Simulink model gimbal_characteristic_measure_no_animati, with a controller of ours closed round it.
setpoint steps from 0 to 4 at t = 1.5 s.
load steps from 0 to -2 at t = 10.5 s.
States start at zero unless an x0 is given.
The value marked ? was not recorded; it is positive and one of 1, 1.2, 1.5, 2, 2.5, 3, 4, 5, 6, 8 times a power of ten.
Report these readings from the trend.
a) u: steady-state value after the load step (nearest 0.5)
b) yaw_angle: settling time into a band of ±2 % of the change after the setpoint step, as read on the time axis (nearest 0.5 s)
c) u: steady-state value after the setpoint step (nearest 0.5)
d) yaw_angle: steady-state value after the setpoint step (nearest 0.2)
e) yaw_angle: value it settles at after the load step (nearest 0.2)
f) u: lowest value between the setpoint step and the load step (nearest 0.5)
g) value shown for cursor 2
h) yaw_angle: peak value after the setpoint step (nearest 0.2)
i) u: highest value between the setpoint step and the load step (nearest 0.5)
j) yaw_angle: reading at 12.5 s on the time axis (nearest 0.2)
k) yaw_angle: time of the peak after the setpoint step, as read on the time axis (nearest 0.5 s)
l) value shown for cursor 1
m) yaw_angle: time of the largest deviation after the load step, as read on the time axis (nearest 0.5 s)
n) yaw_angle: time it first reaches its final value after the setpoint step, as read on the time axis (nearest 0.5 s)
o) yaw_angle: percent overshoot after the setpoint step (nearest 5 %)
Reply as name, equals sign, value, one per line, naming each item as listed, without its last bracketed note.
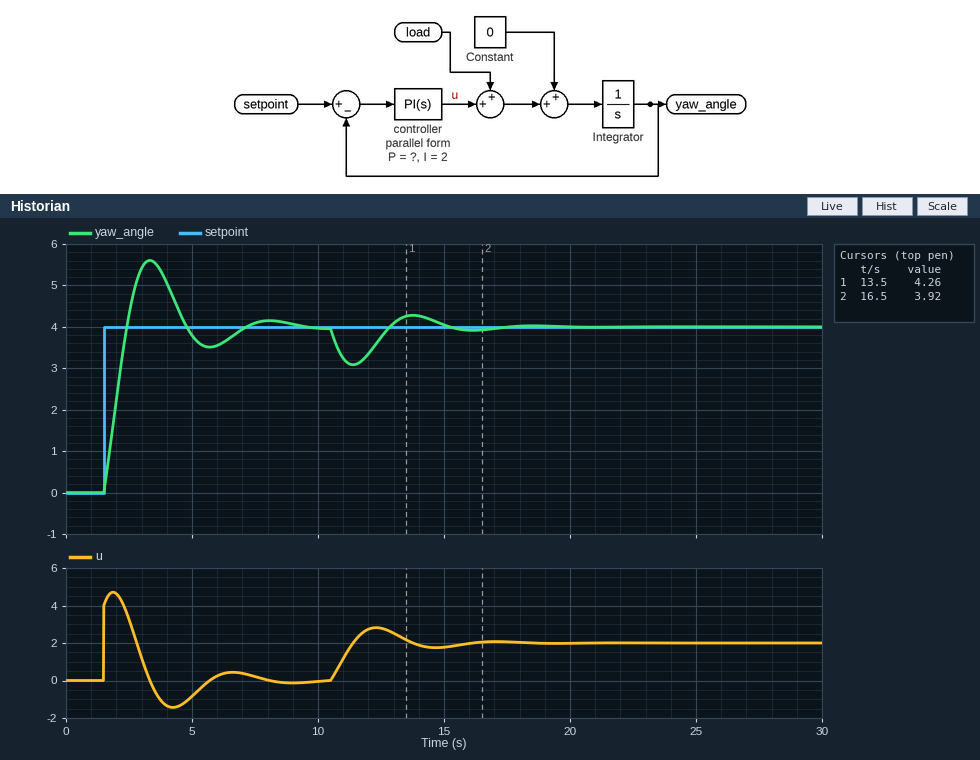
u: steady-state value after the load step = 2.0
yaw_angle: settling time into a band of ±2 % of the change after the setpoint step, as read on the time axis = 9.0 s
u: steady-state value after the setpoint step = 0.0
yaw_angle: steady-state value after the setpoint step = 4.0
yaw_angle: value it settles at after the load step = 4.0
u: lowest value between the setpoint step and the load step = -1.5
value shown for cursor 2 = 3.92
yaw_angle: peak value after the setpoint step = 5.6
u: highest value between the setpoint step and the load step = 4.5
yaw_angle: reading at 12.5 s on the time axis = 3.8
yaw_angle: time of the peak after the setpoint step, as read on the time axis = 3.5 s
value shown for cursor 1 = 4.26
yaw_angle: time of the largest deviation after the load step, as read on the time axis = 11.5 s
yaw_angle: time it first reaches its final value after the setpoint step, as read on the time axis = 2.5 s
yaw_angle: percent overshoot after the setpoint step = 40 %
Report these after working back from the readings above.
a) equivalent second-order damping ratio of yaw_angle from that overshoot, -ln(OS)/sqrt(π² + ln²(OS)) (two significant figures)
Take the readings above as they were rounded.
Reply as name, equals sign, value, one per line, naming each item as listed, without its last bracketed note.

equivalent second-order damping ratio of yaw_angle from that overshoot, -ln(OS)/sqrt(π² + ln²(OS)) = 0.28
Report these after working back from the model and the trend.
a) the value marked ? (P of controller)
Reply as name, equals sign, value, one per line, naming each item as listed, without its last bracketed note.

the value marked ? = 1
